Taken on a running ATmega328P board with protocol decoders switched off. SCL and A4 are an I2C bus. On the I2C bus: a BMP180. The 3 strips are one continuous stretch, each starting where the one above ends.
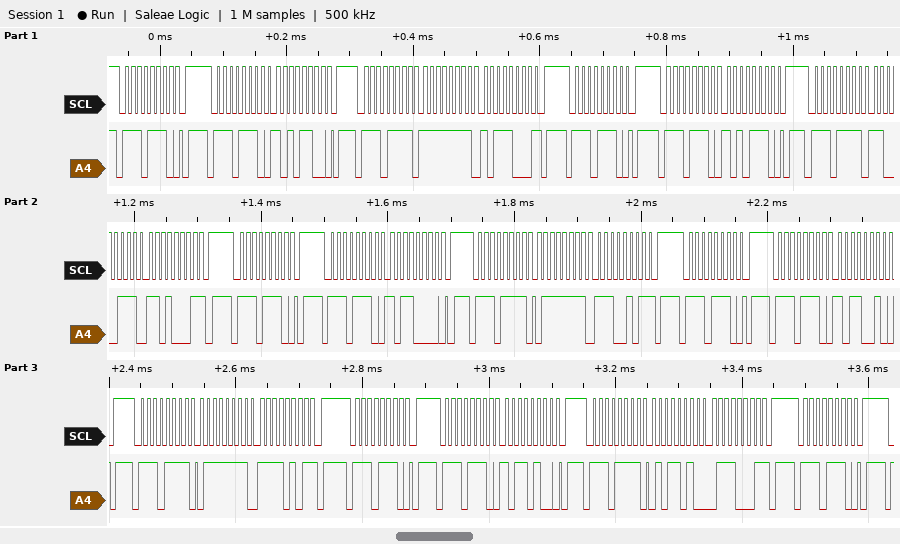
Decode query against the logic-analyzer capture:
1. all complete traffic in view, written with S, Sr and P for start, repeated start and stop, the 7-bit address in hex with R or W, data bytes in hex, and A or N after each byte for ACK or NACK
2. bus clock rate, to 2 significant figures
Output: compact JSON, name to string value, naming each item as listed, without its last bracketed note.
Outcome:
{"all complete traffic in view, written with S, Sr and P for start, repeated start and stop, the 7-bit address in hex with R or W, data bytes in hex, and A or N after each byte for ACK or NACK": "S 77W A P S 77W A AC A P S 77R A FF A B8 N P S 77W A P S 77W A AE A P S 77R A C7 A D1 N P S 77W A P S 77W A B0 A P S 77R A 7F A E5 N P S 77W A P S 77W A B2 A P S 77R A 7F A F5 N P S 77W A P S 77W A B4 A P S 77R A 5A A 71 N P S 77W A P", "bus clock rate, to 2 significant figures": "100 kHz"}
